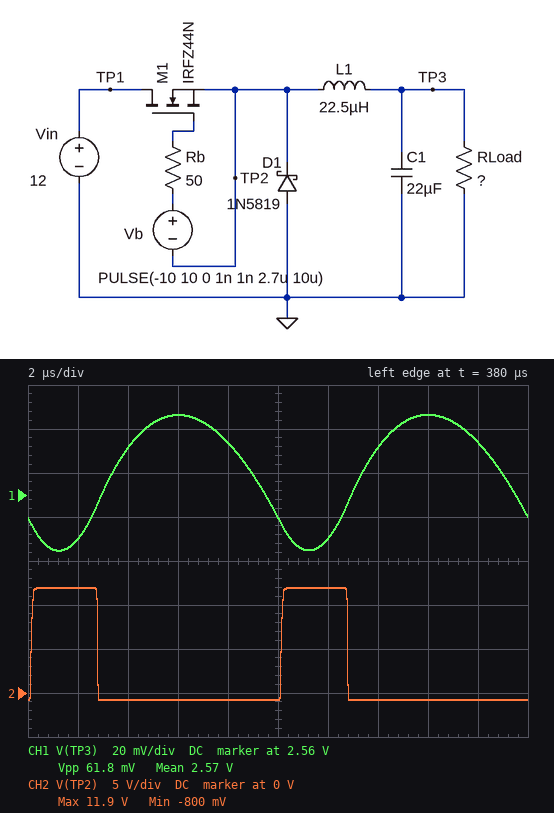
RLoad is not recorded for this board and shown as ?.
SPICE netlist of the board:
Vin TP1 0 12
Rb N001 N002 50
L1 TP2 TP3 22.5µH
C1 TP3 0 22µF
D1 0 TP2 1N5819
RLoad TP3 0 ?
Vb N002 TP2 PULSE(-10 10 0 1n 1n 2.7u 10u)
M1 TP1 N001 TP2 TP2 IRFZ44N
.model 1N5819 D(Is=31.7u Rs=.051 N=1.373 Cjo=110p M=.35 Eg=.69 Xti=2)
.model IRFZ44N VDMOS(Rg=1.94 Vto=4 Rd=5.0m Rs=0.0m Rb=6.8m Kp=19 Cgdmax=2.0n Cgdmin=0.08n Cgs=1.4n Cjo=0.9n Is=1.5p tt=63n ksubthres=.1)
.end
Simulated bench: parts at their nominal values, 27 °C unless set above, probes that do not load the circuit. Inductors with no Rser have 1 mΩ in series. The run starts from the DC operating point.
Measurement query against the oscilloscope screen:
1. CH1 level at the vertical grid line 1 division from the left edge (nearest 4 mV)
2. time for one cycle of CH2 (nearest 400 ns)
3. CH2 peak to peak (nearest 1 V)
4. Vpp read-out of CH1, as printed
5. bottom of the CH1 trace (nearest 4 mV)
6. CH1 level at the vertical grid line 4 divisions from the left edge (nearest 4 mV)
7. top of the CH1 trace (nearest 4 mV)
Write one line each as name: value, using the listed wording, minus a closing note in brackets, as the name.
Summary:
CH1 level at the vertical grid line 1 division from the left edge: 2.540 V
time for one cycle of CH2: 10.0 µs
CH2 peak to peak: 13 V
Vpp read-out of CH1, as printed: 61.8 mV
bottom of the CH1 trace: 2.536 V
CH1 level at the vertical grid line 4 divisions from the left edge: 2.584 V
top of the CH1 trace: 2.596 V
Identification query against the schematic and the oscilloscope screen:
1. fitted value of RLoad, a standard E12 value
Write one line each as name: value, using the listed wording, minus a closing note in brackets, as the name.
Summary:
fitted value of RLoad, a standard E12 value: 0.39 Ω
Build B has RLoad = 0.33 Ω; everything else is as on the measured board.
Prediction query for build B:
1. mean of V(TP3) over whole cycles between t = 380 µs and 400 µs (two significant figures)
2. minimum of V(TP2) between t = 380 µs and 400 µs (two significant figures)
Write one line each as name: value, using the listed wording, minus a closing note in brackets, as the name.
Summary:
mean of V(TP3) over whole cycles between t = 380 µs and 400 µs: 2.5 V
minimum of V(TP2) between t = 380 µs and 400 µs: -860 mV
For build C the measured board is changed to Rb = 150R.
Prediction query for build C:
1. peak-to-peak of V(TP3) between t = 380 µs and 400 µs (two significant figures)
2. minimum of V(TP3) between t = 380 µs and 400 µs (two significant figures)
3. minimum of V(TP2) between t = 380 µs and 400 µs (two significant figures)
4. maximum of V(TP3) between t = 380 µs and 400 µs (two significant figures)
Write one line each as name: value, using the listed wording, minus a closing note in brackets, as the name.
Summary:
peak-to-peak of V(TP3) between t = 380 µs and 400 µs: 60 mV
minimum of V(TP3) between t = 380 µs and 400 µs: 2.4 V
minimum of V(TP2) between t = 380 µs and 400 µs: -780 mV
maximum of V(TP3) between t = 380 µs and 400 µs: 2.5 V
